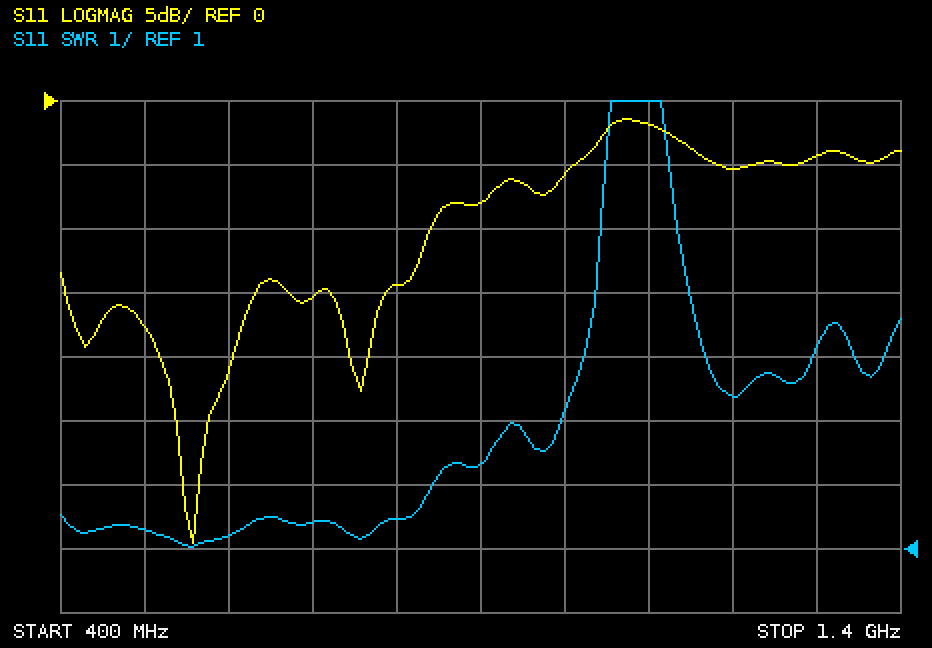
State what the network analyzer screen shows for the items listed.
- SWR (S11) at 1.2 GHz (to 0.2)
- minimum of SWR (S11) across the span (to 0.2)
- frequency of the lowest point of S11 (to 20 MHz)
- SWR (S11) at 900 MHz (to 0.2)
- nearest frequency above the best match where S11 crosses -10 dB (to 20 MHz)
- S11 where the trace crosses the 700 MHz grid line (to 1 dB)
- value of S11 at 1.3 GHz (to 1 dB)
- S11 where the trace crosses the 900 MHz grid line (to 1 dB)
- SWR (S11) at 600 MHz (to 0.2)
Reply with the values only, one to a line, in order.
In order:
3.4
1.0
560 MHz
2.4
840 MHz
-15 dB
-4 dB
-8 dB
1.2
